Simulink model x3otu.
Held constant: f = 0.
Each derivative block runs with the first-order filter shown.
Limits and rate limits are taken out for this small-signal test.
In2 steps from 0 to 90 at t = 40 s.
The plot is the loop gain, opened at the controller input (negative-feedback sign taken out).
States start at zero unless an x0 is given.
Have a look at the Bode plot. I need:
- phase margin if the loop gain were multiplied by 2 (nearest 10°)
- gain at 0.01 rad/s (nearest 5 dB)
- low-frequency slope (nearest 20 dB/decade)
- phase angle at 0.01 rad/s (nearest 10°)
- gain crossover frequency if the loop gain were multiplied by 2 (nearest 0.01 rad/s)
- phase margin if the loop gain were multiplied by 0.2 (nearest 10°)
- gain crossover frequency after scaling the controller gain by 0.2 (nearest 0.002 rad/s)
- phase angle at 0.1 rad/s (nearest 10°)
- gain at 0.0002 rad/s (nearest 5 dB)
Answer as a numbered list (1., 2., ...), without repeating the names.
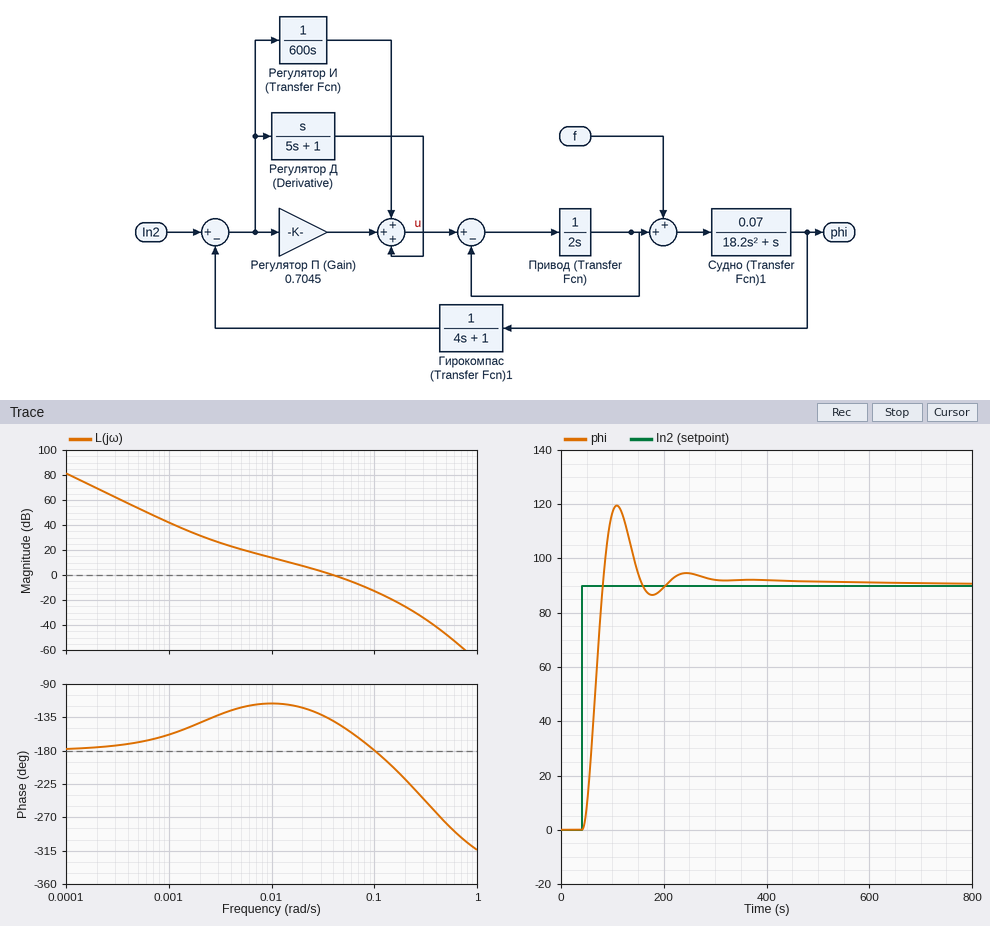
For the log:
1. 20°
2. 15 dB
3. -40 dB/decade
4. -120°
5. 0.06 rad/s
6. 60°
7. 0.010 rad/s
8. -180°
9. 70 dB
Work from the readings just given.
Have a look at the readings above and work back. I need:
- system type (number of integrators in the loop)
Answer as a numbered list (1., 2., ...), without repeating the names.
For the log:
1. 2
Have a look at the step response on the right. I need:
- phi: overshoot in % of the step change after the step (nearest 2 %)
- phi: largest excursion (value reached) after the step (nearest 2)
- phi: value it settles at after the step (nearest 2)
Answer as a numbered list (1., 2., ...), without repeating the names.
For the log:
1. 32 %
2. 120
3. 90
